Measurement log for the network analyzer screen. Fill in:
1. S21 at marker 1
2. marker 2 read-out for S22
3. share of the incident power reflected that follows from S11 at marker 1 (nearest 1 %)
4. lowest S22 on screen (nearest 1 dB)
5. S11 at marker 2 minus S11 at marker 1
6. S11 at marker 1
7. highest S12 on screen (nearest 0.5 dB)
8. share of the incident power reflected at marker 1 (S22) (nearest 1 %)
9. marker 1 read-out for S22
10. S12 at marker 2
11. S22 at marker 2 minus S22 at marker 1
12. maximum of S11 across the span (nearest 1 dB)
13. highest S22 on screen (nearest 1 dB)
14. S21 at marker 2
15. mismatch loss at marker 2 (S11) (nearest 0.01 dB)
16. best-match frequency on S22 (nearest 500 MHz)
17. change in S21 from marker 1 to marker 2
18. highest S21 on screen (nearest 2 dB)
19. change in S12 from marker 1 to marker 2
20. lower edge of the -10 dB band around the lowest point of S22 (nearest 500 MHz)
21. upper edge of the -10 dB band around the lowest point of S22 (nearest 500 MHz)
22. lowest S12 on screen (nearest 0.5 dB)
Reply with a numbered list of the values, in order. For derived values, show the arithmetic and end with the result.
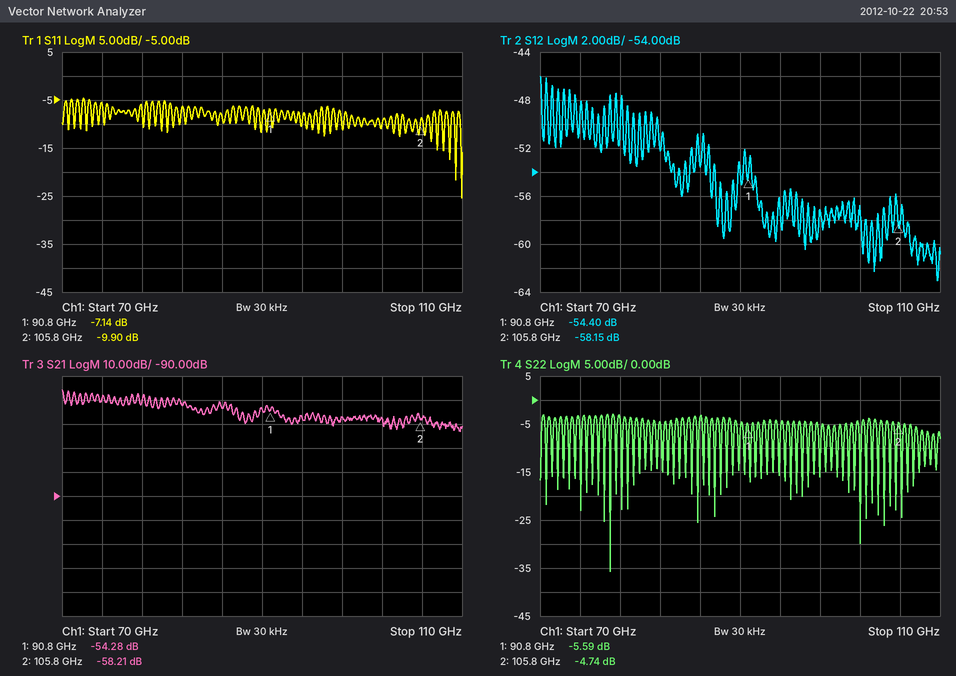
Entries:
1. -54.28 dB
2. -4.74 dB
3. 10^(-7.14/10) ≈ 19 %
4. -36 dB
5. -9.9 − (-7.14) = -2.76 dB
6. -7.14 dB
7. -46.0 dB
8. 10^(-5.59/10) ≈ 28 %
9. -5.59 dB
10. -58.15 dB
11. -4.74 − (-5.59) = 0.85 dB
12. -5 dB
13. -3 dB
14. -58.21 dB
15. −10 log10(1 − 10^(-9.9/10)) ≈ 0.47 dB
16. 77.0 GHz
17. -58.21 − (-54.28) = -3.93 dB
18. -46 dB
19. -58.15 − (-54.4) = -3.75 dB
20. 77.0 GHz
21. 77.0 GHz
22. -63.0 dB
